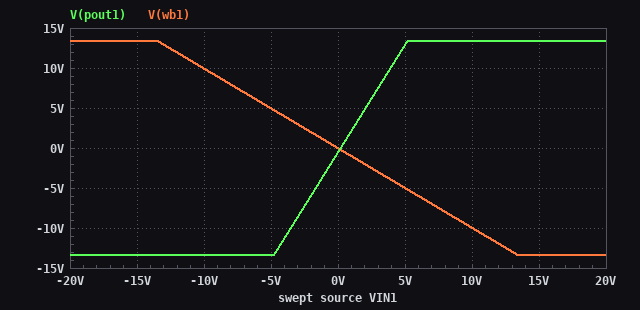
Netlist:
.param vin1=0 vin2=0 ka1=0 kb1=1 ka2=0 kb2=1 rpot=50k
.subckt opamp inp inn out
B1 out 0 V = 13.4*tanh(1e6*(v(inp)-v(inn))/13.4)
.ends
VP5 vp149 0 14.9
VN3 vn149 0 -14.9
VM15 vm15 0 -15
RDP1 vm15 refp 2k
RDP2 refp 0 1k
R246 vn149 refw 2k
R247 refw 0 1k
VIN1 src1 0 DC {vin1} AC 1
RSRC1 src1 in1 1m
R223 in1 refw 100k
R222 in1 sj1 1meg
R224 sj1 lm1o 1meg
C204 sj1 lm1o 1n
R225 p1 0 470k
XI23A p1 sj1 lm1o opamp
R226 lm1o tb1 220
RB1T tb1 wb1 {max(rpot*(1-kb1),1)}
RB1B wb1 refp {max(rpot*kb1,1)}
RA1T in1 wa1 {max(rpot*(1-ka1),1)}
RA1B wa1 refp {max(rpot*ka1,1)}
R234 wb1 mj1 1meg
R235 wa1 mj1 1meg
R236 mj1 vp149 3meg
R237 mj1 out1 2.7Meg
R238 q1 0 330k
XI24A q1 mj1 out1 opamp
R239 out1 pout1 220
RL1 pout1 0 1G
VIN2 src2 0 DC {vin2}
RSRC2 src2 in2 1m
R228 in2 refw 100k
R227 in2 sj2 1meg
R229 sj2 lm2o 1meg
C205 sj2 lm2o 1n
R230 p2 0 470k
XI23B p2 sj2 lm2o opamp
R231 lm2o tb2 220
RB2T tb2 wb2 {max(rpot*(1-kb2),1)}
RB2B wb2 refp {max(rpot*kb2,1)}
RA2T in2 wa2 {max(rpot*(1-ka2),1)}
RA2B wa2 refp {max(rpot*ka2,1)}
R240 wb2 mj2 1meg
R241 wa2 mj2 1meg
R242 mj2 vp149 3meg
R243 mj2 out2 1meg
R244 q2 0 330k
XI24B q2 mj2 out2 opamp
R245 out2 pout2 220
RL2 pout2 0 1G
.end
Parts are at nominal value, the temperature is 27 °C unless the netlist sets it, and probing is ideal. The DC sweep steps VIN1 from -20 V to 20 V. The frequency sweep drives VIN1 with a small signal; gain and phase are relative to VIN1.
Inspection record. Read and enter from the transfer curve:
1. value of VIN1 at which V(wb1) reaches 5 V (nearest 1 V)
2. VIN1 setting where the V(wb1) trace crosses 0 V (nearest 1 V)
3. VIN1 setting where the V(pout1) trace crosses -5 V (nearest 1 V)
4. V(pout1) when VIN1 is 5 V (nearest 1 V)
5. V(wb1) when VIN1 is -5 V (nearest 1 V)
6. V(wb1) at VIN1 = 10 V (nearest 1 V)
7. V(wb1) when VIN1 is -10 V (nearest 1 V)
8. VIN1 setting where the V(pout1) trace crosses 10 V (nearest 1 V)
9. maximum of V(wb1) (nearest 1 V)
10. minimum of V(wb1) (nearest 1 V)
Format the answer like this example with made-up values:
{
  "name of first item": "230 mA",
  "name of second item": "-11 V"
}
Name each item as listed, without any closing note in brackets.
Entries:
{
  "value of VIN1 at which V(wb1) reaches 5 V": "-5 V",
  "VIN1 setting where the V(wb1) trace crosses 0 V": "0 V",
  "VIN1 setting where the V(pout1) trace crosses -5 V": "-2 V",
  "V(pout1) when VIN1 is 5 V": "13 V",
  "V(wb1) when VIN1 is -5 V": "5 V",
  "V(wb1) at VIN1 = 10 V": "-10 V",
  "V(wb1) when VIN1 is -10 V": "10 V",
  "VIN1 setting where the V(pout1) trace crosses 10 V": "4 V",
  "maximum of V(wb1)": "13 V",
  "minimum of V(wb1)": "-13 V"
}
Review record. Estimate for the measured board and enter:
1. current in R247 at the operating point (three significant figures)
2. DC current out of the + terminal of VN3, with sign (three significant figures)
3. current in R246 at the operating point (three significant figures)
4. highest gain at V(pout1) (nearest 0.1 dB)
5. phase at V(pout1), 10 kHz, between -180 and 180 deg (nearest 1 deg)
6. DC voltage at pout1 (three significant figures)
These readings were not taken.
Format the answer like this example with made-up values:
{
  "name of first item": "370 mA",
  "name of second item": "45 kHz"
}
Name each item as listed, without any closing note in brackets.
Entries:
{
  "current in R247 at the operating point": "4.90 mA",
  "DC current out of the + terminal of VN3, with sign": "-5.00 mA",
  "current in R246 at the operating point": "5.00 mA",
  "highest gain at V(pout1)": "8.6 dB",
  "phase at V(pout1), 10 kHz, between -180 and 180 deg": "-128 deg",
  "DC voltage at pout1": "-552 mV"
}
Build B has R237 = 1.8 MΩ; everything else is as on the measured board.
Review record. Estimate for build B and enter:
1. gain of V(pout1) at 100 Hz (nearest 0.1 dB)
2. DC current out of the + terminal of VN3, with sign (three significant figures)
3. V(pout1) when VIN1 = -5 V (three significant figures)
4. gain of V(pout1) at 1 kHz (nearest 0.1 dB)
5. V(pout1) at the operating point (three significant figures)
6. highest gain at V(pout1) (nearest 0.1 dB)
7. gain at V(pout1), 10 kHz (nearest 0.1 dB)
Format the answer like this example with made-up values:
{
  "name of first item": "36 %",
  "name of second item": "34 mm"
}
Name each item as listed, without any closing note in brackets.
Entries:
{
  "gain of V(pout1) at 100 Hz": "3.6 dB",
  "DC current out of the + terminal of VN3, with sign": "-5.00 mA",
  "V(pout1) when VIN1 = -5 V": "-9.33 V",
  "gain of V(pout1) at 1 kHz": "-11.0 dB",
  "V(pout1) at the operating point": "-368 mV",
  "highest gain at V(pout1)": "5.1 dB",
  "gain at V(pout1), 10 kHz": "-28.7 dB"
}
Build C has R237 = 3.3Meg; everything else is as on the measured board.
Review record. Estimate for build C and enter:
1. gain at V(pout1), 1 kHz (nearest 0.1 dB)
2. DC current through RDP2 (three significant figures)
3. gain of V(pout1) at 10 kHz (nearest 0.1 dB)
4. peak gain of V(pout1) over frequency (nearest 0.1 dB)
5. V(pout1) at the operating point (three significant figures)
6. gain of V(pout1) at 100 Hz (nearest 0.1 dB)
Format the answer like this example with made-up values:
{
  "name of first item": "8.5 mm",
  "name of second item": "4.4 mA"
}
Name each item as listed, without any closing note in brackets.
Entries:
{
  "gain at V(pout1), 1 kHz": "-5.7 dB",
  "DC current through RDP2": "4.74 mA",
  "gain of V(pout1) at 10 kHz": "-23.5 dB",
  "peak gain of V(pout1) over frequency": "10.3 dB",
  "V(pout1) at the operating point": "-675 mV",
  "gain of V(pout1) at 100 Hz": "8.9 dB"
}
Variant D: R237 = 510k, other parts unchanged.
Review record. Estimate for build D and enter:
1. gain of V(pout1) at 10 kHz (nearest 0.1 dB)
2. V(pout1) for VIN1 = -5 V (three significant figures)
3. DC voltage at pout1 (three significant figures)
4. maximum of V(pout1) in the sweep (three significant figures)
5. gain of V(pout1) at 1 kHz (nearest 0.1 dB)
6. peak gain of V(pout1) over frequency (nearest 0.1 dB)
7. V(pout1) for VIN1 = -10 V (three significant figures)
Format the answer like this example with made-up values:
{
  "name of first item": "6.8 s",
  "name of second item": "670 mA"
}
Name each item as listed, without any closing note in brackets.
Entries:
{
  "gain of V(pout1) at 10 kHz": "-39.7 dB",
  "V(pout1) for VIN1 = -5 V": "-2.64 V",
  "DC voltage at pout1": "-104 mV",
  "maximum of V(pout1) in the sweep": "6.70 V",
  "gain of V(pout1) at 1 kHz": "-21.9 dB",
  "peak gain of V(pout1) over frequency": "-5.9 dB",
  "V(pout1) for VIN1 = -10 V": "-5.18 V"
}
